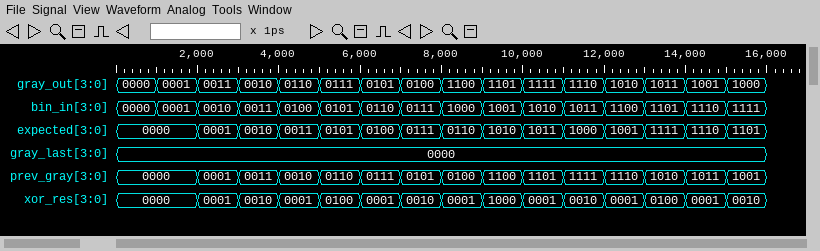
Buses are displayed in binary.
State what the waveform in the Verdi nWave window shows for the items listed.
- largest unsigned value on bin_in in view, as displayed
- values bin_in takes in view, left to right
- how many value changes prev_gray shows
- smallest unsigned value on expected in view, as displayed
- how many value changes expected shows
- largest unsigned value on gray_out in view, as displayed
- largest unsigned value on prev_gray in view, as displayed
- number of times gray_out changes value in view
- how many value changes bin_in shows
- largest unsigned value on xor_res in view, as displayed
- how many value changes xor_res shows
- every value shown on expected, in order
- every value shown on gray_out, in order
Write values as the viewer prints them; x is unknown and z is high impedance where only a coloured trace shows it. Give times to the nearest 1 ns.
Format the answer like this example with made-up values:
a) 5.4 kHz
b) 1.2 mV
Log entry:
a) 1111
b) 0000, 0001, 0010, 0011, 0100, 0101, 0110, 0111, 1000, 1001, 1010, 1011, 1100, 1101, 1110, 1111
c) 14
d) 0000
e) 14
f) 1111
g) 1111
h) 15
i) 15
j) 1000
k) 14
l) 0000, 0001, 0010, 0011, 0101, 0100, 0111, 0110, 1010, 1011, 1000, 1001, 1111, 1110, 1101
m) 0000, 0001, 0011, 0010, 0110, 0111, 0101, 0100, 1100, 1101, 1111, 1110, 1010, 1011, 1001, 1000
